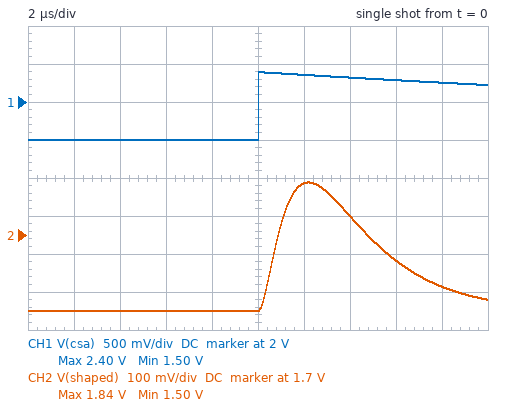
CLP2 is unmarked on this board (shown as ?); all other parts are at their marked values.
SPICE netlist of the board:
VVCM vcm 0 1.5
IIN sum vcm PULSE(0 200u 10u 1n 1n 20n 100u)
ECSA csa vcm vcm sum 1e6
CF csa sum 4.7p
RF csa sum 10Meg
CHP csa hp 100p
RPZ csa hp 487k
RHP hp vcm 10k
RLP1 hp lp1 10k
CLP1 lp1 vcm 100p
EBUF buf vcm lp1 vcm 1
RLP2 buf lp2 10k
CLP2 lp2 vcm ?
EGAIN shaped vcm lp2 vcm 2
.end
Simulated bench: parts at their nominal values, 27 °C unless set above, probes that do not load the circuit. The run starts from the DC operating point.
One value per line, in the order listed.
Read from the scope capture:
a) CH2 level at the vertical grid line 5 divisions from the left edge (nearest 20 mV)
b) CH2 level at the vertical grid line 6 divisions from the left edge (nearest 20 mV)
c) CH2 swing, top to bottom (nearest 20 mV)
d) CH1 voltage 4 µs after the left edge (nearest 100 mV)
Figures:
1.50 V
1.84 V
340 mV
1.5 V
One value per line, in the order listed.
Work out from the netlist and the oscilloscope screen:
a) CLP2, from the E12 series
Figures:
120 pF
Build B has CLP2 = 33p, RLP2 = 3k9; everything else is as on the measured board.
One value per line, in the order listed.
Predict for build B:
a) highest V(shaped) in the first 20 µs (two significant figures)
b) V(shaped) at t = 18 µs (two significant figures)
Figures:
2.0 V
1.5 V
